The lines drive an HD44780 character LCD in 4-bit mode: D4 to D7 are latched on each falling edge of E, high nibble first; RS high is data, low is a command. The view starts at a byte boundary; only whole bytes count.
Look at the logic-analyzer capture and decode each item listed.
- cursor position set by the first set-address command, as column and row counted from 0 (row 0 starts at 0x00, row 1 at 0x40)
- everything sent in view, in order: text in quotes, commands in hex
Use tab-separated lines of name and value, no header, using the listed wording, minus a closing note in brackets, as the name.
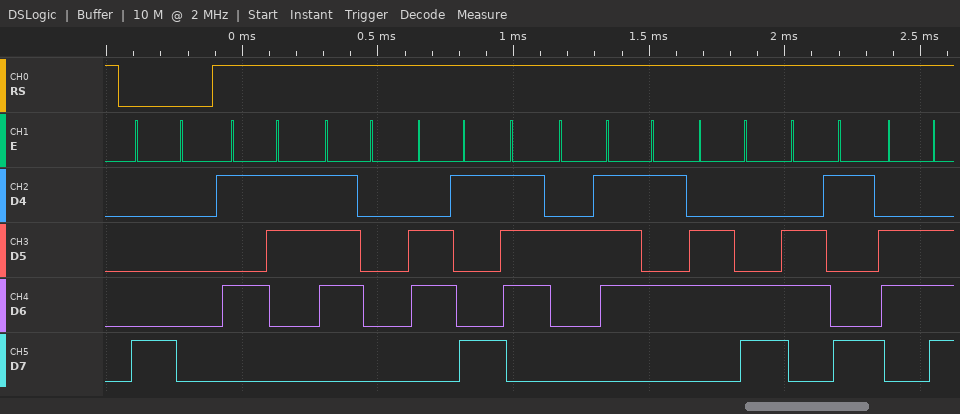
cursor position set by the first set-address command, as column and row counted from 0	column 0, row 0
everything sent in view, in order: text in quotes, commands in hex	0x80 "Spirulin"
